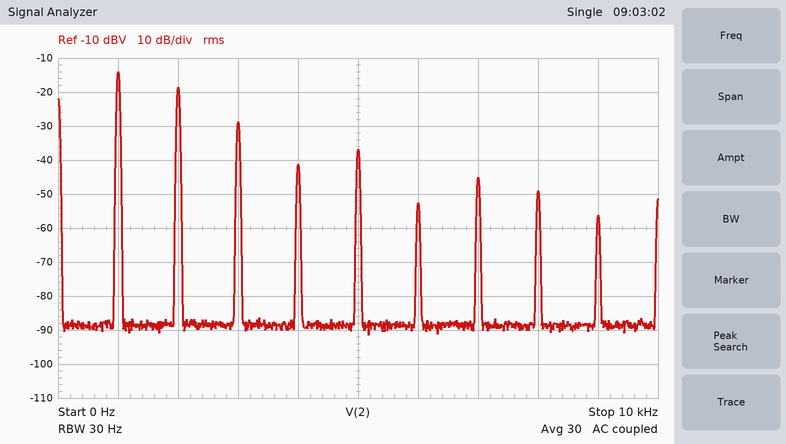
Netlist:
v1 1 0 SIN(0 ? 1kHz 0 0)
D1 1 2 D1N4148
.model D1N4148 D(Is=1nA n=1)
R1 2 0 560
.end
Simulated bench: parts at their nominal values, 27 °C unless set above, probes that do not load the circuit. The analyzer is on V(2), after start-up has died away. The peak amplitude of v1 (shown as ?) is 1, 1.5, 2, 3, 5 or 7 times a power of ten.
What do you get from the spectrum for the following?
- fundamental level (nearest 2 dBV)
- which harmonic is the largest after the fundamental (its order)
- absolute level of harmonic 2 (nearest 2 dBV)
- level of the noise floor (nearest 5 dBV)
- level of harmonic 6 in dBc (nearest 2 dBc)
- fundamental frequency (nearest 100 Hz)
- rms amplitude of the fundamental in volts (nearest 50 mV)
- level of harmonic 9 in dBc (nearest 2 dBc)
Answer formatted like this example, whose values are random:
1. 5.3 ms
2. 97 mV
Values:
1. -14 dBV
2. 2
3. -18 dBV
4. -90 dBV
5. -38 dBc
6. 1.0 kHz
7. 200 mV
8. -42 dBc
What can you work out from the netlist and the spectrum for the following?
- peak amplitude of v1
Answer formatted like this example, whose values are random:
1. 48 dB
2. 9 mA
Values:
1. 1 V
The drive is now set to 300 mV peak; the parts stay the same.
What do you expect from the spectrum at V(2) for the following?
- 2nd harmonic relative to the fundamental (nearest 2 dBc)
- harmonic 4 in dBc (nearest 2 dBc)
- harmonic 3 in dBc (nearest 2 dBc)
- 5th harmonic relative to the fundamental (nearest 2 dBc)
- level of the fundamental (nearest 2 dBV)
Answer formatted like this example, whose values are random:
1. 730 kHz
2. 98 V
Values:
1. -2 dBc
2. -8 dBc
3. -4 dBc
4. -14 dBc
5. -46 dBV
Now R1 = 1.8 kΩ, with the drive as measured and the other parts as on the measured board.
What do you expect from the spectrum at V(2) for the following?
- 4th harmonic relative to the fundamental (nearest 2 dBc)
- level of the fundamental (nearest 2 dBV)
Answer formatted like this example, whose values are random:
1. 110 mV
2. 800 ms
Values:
1. -26 dBc
2. -14 dBV
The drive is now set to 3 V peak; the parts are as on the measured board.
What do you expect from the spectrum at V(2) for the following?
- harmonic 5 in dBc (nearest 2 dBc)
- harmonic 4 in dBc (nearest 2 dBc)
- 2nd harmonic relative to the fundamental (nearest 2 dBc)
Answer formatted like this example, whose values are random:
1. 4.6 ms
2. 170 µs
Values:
1. -30 dBc
2. -22 dBc
3. -6 dBc
